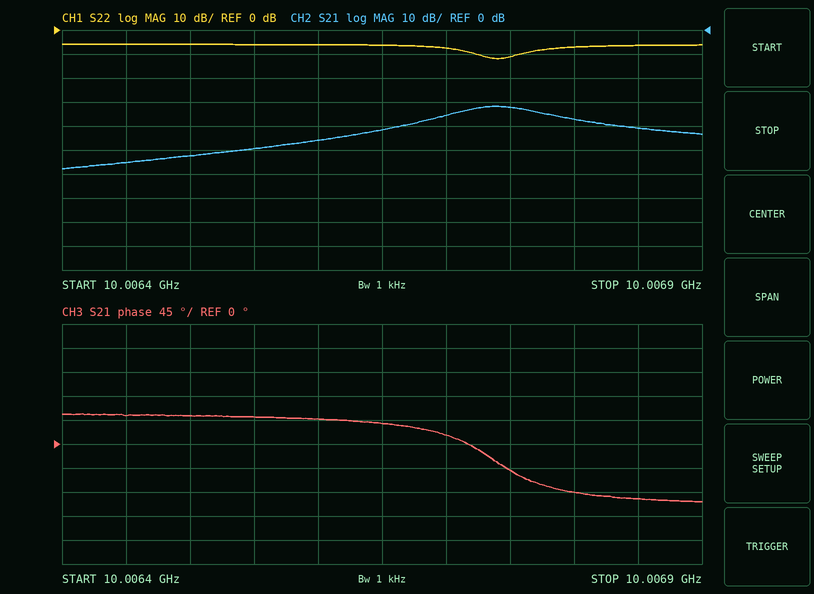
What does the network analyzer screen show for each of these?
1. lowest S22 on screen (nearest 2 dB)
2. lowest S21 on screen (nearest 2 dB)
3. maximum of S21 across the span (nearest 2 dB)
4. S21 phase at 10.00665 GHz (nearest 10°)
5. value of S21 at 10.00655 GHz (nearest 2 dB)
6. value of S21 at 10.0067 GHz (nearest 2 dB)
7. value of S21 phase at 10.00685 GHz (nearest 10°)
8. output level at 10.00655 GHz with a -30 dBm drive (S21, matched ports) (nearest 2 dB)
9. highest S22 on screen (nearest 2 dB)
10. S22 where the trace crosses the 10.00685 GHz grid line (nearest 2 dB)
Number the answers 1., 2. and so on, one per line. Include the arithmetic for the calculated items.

1. -12 dB
2. -58 dB
3. -32 dB
4. 40°
5. -50 dB
6. -36 dB
7. -100°
8. -30 dBm + (-50 dB) = -80 dBm
9. -6 dB
10. -6 dB
